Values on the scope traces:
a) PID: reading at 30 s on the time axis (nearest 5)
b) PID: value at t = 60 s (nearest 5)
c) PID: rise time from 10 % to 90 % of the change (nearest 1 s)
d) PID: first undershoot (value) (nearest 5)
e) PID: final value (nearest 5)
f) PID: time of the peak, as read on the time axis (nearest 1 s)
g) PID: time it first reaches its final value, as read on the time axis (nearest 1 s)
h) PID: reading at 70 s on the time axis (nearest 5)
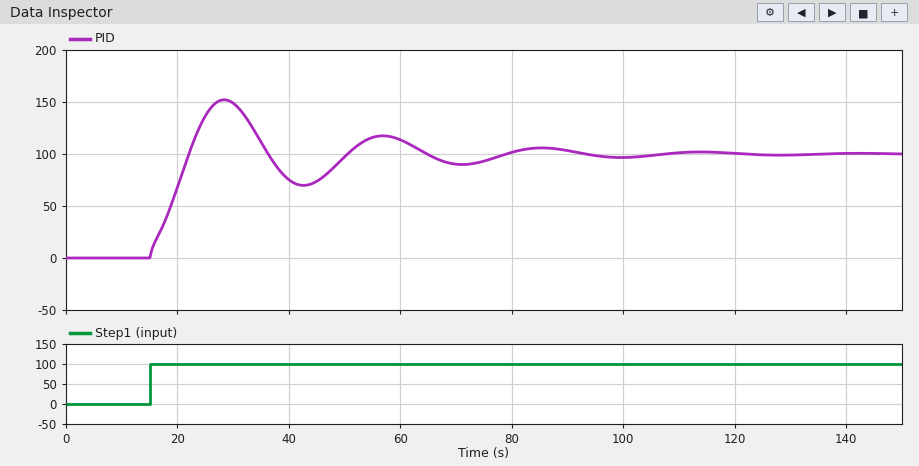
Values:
150
115
6 s
70
100
28 s
22 s
90
